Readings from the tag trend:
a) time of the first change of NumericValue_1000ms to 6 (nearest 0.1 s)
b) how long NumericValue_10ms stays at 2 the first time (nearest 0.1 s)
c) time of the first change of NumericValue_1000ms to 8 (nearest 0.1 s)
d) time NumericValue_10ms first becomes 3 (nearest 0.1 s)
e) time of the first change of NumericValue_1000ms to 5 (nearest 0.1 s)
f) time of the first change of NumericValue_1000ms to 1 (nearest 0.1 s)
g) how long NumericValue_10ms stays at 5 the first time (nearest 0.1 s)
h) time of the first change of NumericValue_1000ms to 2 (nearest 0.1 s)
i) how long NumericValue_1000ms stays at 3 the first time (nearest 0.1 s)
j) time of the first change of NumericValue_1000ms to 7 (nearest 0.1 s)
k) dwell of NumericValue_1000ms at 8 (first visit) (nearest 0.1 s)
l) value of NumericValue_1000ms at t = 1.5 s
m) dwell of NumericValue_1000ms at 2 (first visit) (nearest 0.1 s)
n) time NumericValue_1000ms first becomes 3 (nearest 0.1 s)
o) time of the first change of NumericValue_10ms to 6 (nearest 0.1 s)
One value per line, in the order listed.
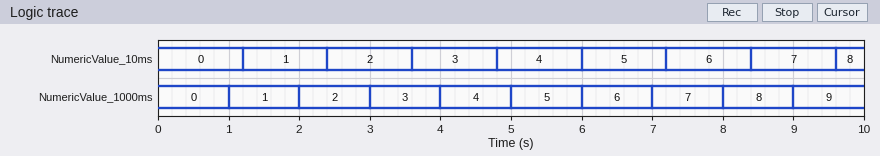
6.0 s
1.2 s
8.0 s
3.6 s
5.0 s
1.0 s
1.2 s
2.0 s
1.0 s
7.0 s
1.0 s
1
1.0 s
3.0 s
7.2 s
